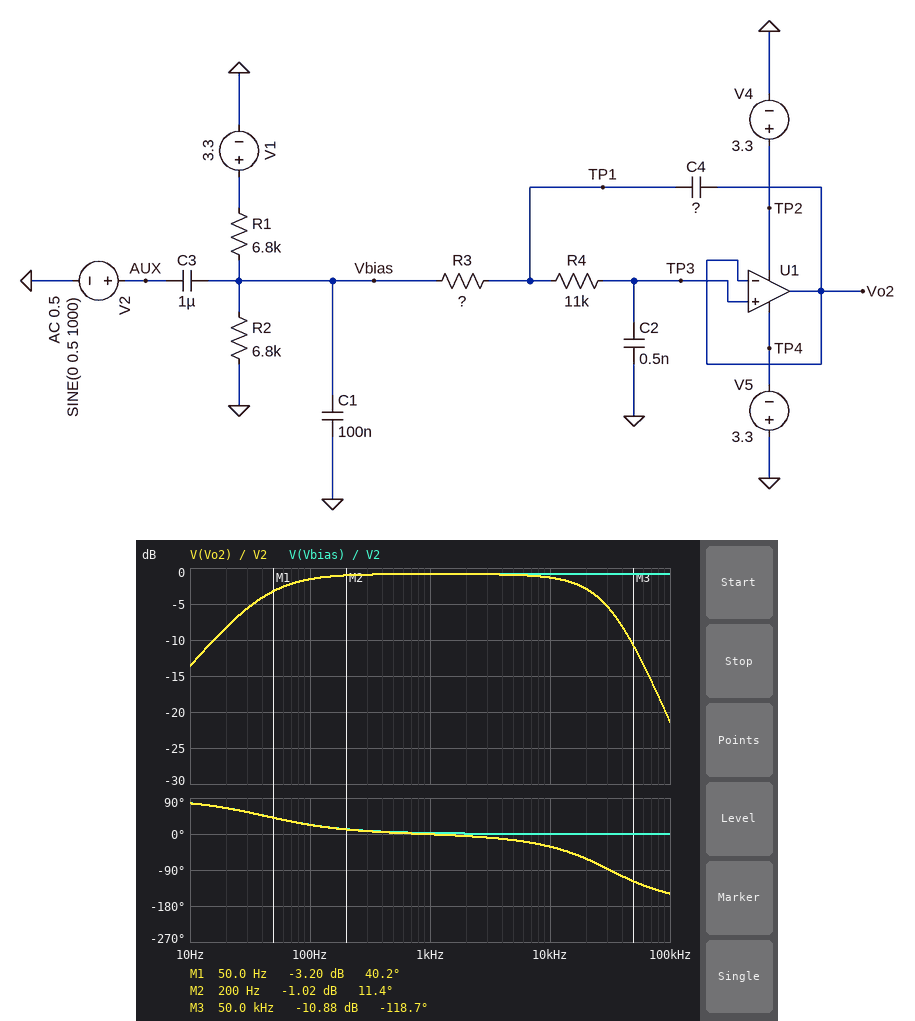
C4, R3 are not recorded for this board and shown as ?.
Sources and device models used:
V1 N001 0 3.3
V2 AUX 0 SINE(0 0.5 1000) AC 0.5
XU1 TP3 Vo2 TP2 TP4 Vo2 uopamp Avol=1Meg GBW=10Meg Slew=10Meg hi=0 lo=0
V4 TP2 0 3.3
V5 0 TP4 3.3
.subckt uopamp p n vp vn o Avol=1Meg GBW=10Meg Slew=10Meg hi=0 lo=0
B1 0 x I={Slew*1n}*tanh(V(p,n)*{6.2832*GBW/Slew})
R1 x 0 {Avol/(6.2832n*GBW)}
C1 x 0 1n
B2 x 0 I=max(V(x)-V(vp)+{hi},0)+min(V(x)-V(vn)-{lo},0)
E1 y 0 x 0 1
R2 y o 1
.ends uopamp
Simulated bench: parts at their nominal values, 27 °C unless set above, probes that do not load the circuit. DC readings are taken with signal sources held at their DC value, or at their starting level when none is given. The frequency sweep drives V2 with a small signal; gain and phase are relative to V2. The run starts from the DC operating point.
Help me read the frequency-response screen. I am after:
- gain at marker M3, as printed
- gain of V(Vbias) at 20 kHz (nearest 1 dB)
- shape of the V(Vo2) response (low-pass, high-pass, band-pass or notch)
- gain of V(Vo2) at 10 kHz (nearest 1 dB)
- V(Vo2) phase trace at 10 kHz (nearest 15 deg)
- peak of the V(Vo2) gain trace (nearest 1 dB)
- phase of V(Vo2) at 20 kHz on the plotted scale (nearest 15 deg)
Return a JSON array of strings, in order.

["-10.88 dB", "-1 dB", "band-pass", "-1 dB", "-30 deg", "-1 dB", "-60 deg"]
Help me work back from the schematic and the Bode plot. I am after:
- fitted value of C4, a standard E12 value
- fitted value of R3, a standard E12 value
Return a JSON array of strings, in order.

["680 pF", "6.8 kΩ"]
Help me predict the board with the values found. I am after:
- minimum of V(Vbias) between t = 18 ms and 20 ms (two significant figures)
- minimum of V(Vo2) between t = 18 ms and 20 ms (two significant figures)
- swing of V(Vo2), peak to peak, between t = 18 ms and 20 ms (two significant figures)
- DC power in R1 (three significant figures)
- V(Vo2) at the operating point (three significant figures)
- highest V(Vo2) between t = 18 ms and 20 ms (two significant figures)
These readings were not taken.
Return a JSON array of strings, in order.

["1.2 V", "1.2 V", "910 mV", "400 µW", "1.65 V", "2.1 V"]
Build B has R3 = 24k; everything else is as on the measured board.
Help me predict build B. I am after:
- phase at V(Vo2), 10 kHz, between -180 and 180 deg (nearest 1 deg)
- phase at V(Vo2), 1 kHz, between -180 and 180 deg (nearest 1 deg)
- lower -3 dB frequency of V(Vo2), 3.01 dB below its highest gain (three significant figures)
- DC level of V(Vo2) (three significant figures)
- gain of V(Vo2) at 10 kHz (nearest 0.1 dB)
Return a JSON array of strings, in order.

["-59 deg", "-4 deg", "42.3 Hz", "1.65 V", "-2.9 dB"]
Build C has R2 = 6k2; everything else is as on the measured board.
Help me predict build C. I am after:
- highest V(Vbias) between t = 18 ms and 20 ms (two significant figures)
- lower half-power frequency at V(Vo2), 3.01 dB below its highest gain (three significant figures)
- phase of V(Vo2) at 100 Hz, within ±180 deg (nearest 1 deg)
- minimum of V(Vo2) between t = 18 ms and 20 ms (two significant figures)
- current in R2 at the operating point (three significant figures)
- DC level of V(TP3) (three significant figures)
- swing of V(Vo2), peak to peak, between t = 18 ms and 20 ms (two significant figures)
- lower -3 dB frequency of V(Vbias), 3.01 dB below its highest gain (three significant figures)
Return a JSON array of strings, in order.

["2.0 V", "44.5 Hz", "24 deg", "1.1 V", "254 µA", "1.57 V", "910 mV", "44.6 Hz"]
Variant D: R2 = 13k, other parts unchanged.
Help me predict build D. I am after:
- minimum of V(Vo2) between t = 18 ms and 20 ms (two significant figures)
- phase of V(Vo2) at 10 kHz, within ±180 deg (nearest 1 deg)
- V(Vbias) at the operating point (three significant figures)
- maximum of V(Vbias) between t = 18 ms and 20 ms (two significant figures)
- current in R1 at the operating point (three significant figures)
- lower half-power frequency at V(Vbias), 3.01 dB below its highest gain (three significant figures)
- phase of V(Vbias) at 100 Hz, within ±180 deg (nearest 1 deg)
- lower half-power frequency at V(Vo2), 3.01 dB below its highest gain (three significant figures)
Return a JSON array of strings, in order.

["1.7 V", "-32 deg", "2.17 V", "2.6 V", "167 µA", "32.4 Hz", "18 deg", "32.3 Hz"]
